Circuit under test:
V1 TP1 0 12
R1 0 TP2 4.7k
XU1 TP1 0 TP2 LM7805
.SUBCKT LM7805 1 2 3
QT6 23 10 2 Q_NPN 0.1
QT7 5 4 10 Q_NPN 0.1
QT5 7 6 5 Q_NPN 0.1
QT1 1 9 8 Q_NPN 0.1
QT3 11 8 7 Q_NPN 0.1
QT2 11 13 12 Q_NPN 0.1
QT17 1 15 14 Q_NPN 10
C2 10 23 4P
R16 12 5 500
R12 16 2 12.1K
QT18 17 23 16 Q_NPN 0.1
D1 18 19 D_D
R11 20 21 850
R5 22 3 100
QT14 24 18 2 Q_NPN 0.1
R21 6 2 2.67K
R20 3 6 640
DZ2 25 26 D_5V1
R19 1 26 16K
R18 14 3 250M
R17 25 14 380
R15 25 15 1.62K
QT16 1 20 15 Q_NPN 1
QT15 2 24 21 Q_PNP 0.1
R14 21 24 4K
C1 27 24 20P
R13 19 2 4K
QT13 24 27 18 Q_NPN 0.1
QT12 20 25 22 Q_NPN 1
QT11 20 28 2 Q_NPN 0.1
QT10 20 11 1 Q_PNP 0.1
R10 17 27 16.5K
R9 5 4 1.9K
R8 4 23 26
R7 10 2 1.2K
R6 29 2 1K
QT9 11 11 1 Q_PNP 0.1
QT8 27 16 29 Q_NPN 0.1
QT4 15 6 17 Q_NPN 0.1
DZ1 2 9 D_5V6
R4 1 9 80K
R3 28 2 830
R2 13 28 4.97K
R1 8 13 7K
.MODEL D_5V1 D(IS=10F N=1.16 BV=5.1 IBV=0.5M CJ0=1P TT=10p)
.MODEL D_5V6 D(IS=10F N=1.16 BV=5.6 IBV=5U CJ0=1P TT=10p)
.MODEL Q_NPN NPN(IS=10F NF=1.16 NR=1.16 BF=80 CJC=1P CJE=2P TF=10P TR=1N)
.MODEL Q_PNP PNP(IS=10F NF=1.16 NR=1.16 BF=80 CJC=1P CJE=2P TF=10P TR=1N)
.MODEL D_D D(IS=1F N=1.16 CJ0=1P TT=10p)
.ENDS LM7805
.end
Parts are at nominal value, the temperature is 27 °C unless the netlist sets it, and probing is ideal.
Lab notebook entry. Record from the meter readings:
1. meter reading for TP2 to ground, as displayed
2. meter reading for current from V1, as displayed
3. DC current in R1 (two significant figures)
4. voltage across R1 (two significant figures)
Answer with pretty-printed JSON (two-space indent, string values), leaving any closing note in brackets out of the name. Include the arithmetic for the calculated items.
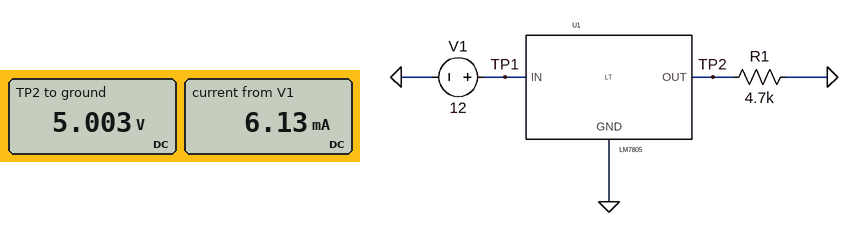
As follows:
{
  "meter reading for TP2 to ground, as displayed": "5.003 V",
  "meter reading for current from V1, as displayed": "6.13 mA",
  "DC current in R1": "(5.003 V) / 4.7 kΩ = 1.1 mA",
  "voltage across R1": "5.003 V = 5.0 V"
}
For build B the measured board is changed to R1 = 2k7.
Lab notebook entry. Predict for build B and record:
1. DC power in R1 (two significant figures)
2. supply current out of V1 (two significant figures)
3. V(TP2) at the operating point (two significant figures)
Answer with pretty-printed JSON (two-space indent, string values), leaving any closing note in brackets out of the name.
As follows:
{
  "DC power in R1": "9.3 mW",
  "supply current out of V1": "6.9 mA",
  "V(TP2) at the operating point": "5.0 V"
}
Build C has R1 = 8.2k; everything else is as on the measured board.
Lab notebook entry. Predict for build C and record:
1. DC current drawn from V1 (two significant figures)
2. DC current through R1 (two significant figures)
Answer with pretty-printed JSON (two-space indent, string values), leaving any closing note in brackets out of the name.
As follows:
{
  "DC current drawn from V1": "5.7 mA",
  "DC current through R1": "610 µA"
}
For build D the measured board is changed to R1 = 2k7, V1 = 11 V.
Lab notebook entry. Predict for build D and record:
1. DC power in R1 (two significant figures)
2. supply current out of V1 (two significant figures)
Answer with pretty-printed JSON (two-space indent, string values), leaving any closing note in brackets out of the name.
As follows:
{
  "DC power in R1": "9.3 mW",
  "supply current out of V1": "6.9 mA"
}
